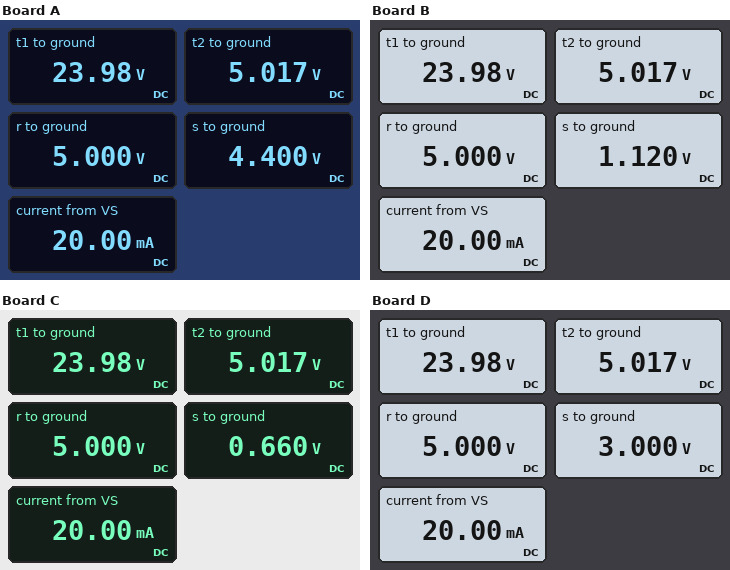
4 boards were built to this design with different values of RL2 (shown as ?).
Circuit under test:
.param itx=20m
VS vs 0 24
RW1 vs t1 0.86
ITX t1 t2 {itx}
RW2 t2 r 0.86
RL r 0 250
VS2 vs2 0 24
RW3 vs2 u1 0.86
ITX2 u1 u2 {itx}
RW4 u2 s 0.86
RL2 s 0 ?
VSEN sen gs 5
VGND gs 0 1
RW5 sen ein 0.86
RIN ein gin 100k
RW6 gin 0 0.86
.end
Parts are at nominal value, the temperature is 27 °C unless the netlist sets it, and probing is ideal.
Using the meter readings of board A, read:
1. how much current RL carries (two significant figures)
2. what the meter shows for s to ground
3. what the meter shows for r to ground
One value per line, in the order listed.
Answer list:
20 mA
4.400 V
5.000 V
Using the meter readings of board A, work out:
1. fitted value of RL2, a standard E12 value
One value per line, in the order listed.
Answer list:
220 Ω
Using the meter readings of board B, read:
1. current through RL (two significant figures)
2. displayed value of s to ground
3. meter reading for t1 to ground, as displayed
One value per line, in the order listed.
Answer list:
20 mA
1.120 V
23.98 V
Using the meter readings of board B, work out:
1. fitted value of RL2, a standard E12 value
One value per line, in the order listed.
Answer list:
56 Ω
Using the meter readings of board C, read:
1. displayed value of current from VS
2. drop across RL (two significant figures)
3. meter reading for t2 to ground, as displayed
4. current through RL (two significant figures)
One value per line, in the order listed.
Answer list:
20.00 mA
5.0 V
5.017 V
20 mA
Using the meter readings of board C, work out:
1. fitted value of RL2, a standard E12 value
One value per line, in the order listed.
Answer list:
33 Ω
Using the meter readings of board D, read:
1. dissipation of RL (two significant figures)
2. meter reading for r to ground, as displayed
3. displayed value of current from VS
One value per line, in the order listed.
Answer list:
100 mW
5.000 V
20.00 mA
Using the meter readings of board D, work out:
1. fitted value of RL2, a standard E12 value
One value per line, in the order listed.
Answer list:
150 Ω
